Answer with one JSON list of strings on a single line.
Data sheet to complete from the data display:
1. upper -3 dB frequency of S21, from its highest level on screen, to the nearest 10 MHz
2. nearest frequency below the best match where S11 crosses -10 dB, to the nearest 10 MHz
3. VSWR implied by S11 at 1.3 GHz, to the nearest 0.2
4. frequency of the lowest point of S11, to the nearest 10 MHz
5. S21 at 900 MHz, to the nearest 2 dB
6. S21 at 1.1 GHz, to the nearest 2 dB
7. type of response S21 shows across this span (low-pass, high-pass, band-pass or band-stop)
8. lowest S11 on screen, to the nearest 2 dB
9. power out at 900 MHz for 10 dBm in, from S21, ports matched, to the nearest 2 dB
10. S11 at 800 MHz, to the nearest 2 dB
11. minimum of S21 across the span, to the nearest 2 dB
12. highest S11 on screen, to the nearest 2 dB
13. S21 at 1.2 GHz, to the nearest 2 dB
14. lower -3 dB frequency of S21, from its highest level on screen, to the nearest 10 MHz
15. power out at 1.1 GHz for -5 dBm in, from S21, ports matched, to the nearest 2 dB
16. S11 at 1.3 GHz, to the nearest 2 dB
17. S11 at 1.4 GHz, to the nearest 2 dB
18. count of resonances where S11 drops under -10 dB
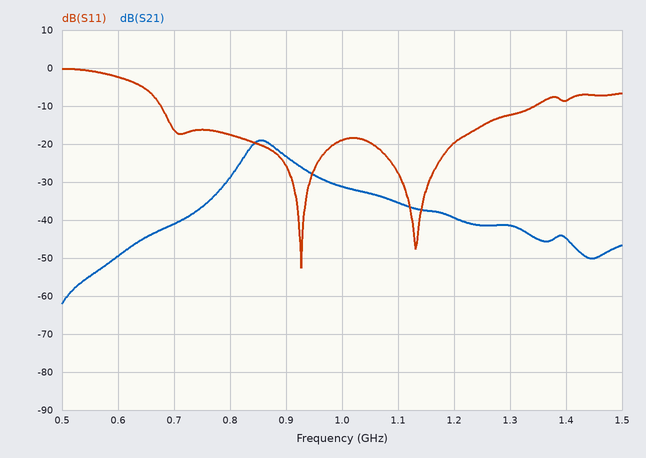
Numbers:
["890 MHz", "680 MHz", "1.6", "930 MHz", "-24 dB", "-36 dB", "band-pass", "-52 dB", "-14 dBm", "-18 dB", "-62 dB", "0 dB", "-40 dB", "830 MHz", "-40 dBm", "-12 dB", "-8 dB", "2"]
